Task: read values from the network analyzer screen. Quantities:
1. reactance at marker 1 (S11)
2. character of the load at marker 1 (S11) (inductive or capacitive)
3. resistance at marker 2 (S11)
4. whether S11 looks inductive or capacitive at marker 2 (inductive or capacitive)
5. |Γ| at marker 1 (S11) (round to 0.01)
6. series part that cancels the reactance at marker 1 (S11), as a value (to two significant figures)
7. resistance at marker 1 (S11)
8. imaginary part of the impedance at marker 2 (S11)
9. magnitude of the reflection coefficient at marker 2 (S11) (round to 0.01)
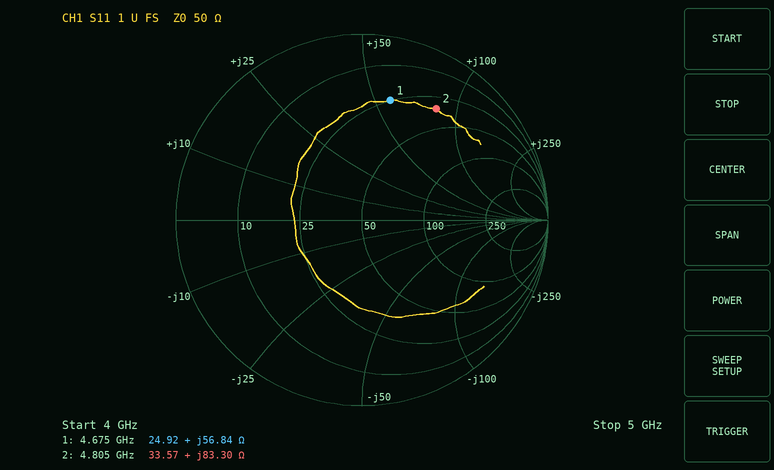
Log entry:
+56.84 Ω
inductive
33.57 Ω
inductive
0.66
600 fF
24.92 Ω
+83.30 Ω
0.72
